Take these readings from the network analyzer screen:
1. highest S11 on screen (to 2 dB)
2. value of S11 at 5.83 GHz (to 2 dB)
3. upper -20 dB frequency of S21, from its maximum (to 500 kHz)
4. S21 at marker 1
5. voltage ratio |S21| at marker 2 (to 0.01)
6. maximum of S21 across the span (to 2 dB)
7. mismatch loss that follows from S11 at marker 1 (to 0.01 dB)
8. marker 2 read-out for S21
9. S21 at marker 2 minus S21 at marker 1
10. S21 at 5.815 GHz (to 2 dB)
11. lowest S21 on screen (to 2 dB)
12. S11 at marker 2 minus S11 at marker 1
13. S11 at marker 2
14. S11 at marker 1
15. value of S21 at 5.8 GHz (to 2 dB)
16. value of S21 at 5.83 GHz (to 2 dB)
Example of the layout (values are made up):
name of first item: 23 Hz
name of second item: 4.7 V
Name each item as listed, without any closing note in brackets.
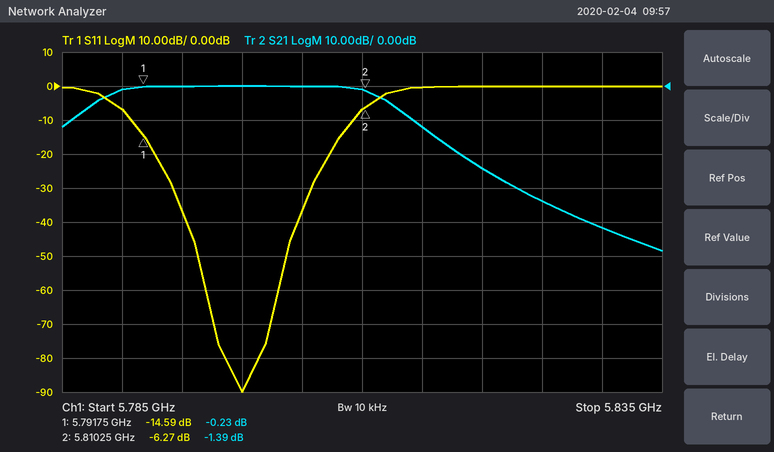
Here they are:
highest S11 on screen: 0 dB
value of S11 at 5.83 GHz: 0 dB
upper -20 dB frequency of S21, from its maximum: 5.8180 GHz
S21 at marker 1: -0.23 dB
voltage ratio |S21| at marker 2: 0.85
maximum of S21 across the span: 0 dB
mismatch loss that follows from S11 at marker 1: 0.15 dB
marker 2 read-out for S21: -1.39 dB
S21 at marker 2 minus S21 at marker 1: -1.16 dB
S21 at 5.815 GHz: -12 dB
lowest S21 on screen: -48 dB
S11 at marker 2 minus S11 at marker 1: 8.32 dB
S11 at marker 2: -6.27 dB
S11 at marker 1: -14.59 dB
value of S21 at 5.8 GHz: 0 dB
value of S21 at 5.83 GHz: -42 dB
